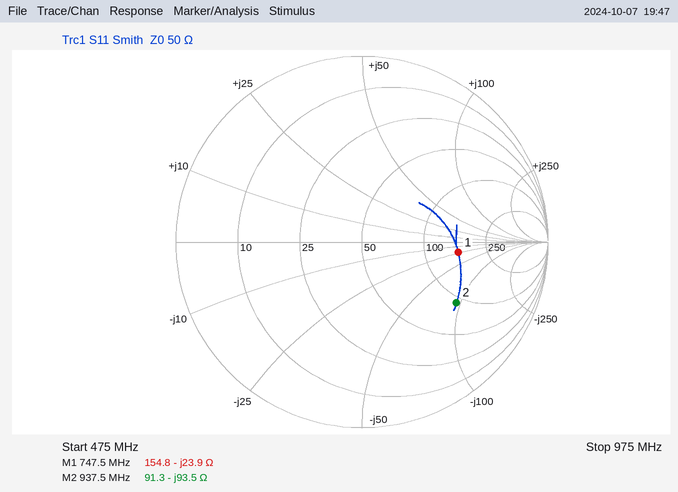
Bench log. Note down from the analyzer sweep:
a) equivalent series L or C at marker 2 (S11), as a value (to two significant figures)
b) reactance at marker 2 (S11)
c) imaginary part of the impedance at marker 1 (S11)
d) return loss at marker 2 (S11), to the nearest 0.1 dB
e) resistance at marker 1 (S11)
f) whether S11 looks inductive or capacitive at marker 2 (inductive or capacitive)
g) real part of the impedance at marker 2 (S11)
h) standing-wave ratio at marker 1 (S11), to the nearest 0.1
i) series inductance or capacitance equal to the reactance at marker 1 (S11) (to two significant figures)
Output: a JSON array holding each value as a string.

["1.8 pF", "-93.5 Ω", "-23.9 Ω", "4.4 dB", "154.8 Ω", "capacitive", "91.3 Ω", "3.2", "8.9 pF"]
